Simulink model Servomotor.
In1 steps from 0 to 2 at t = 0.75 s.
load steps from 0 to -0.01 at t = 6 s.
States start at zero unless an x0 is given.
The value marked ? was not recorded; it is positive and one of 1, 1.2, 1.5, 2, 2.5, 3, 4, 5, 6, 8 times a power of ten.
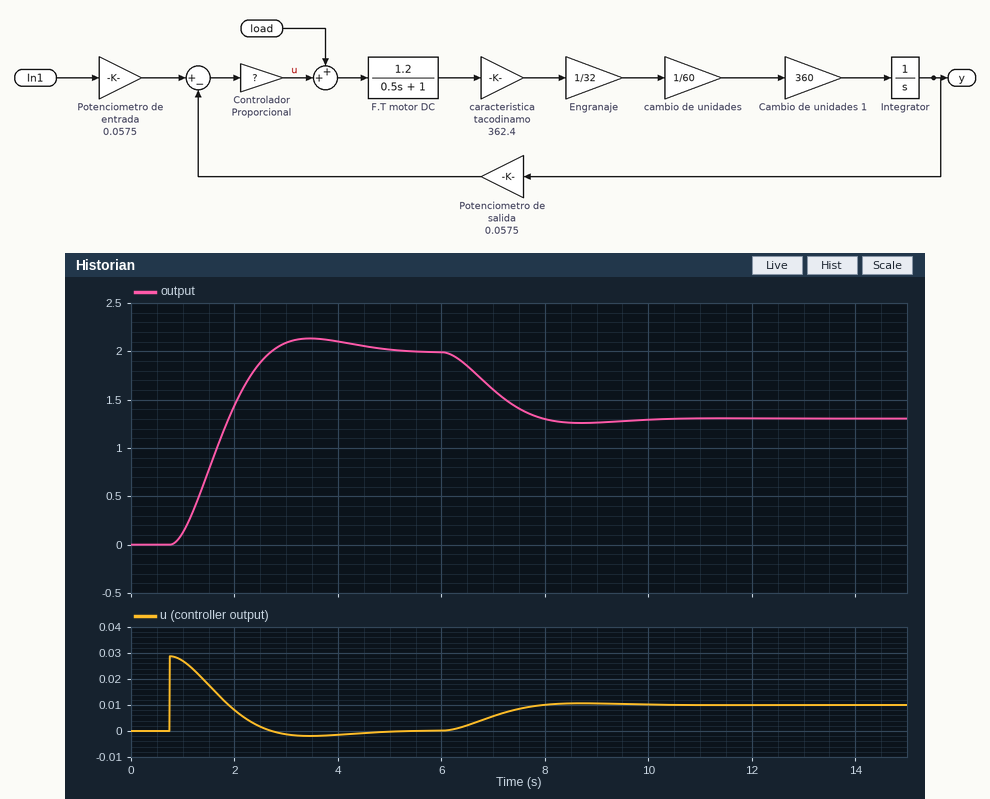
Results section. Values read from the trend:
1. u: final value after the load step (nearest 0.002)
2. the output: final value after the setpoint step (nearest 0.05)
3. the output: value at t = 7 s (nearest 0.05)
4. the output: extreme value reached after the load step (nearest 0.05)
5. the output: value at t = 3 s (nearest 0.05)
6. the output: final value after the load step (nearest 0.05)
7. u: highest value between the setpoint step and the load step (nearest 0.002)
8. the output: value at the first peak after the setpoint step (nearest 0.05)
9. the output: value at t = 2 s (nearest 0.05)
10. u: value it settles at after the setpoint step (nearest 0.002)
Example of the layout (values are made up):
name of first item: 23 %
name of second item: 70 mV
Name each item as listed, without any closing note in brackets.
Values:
u: final value after the load step: 0.010
the output: final value after the setpoint step: 2.00
the output: value at t = 7 s: 1.60
the output: extreme value reached after the load step: 1.25
the output: value at t = 3 s: 2.10
the output: final value after the load step: 1.30
u: highest value between the setpoint step and the load step: 0.028
the output: value at the first peak after the setpoint step: 2.15
the output: value at t = 2 s: 1.45
u: value it settles at after the setpoint step: 0.000
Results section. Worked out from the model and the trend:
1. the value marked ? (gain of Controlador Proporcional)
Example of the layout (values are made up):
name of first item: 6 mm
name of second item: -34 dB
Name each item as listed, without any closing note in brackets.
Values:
the value marked ?: 0.25
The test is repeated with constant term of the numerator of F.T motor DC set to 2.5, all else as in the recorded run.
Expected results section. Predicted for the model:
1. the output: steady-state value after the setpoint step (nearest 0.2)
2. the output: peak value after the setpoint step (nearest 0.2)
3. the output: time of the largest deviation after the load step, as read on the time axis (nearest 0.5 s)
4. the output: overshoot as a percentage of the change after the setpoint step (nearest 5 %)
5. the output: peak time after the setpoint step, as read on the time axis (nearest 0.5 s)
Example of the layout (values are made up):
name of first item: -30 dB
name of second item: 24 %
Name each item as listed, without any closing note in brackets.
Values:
the output: steady-state value after the setpoint step: 2.0
the output: peak value after the setpoint step: 2.4
the output: time of the largest deviation after the load step, as read on the time axis: 7.5 s
the output: overshoot as a percentage of the change after the setpoint step: 20 %
the output: peak time after the setpoint step, as read on the time axis: 2.5 s
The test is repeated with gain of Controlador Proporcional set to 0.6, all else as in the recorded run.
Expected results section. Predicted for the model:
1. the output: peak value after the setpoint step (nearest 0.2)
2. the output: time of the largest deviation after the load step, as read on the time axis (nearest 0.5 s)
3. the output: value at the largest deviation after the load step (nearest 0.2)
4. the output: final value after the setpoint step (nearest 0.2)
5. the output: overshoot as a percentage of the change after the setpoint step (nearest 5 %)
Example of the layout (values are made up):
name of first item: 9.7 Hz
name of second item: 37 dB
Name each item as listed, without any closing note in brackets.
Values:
the output: peak value after the setpoint step: 2.4
the output: time of the largest deviation after the load step, as read on the time axis: 7.5 s
the output: value at the largest deviation after the load step: 1.6
the output: final value after the setpoint step: 2.0
the output: overshoot as a percentage of the change after the setpoint step: 25 %
